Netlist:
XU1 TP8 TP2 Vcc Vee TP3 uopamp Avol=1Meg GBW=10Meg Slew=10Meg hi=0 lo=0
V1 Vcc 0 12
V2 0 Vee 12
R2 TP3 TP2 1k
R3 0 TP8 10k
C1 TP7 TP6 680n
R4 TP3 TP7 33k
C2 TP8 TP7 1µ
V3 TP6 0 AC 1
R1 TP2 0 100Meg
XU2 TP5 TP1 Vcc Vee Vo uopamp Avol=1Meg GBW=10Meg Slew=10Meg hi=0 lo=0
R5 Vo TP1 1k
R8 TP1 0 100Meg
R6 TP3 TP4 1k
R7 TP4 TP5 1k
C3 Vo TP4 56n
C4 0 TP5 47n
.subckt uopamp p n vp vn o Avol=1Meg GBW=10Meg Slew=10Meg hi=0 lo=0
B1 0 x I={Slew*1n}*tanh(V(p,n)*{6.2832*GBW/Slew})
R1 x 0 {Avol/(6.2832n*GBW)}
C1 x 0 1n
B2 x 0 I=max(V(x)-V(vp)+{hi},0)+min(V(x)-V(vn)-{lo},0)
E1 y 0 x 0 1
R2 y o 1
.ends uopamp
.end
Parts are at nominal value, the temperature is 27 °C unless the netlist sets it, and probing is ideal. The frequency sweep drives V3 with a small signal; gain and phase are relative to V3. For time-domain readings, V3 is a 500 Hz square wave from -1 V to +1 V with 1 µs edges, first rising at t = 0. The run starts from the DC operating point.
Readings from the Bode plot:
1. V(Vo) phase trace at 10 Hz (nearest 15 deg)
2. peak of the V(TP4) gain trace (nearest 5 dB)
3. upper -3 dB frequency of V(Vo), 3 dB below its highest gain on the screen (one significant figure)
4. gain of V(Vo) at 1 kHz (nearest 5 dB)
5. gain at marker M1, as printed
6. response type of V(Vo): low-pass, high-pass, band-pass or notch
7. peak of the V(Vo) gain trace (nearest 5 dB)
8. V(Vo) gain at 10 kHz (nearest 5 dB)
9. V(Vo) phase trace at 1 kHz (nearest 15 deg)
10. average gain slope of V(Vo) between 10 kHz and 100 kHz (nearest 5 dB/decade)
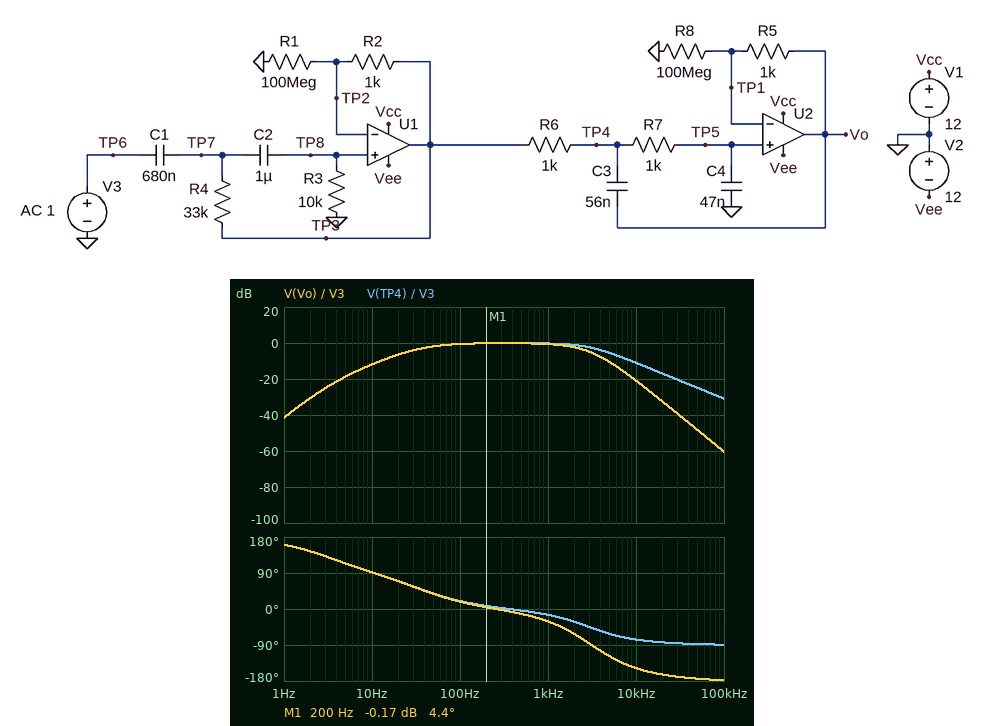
90 deg
0 dB
2 kHz
0 dB
-0.17 dB
band-pass
0 dB
-20 dB
-30 deg
-40 dB/decade
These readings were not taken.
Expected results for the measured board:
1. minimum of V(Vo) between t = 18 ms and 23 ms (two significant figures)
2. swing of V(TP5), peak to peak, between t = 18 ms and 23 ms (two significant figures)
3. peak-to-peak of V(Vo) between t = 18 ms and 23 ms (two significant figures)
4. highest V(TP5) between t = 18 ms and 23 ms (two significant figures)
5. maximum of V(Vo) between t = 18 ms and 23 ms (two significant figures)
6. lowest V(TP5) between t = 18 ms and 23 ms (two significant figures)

-1.1 V
2.1 V
2.1 V
1.0 V
1.0 V
-1.1 V
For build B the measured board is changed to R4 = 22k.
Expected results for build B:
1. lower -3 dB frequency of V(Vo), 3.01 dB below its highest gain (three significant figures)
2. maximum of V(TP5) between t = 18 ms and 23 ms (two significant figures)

34.2 Hz
990 mV
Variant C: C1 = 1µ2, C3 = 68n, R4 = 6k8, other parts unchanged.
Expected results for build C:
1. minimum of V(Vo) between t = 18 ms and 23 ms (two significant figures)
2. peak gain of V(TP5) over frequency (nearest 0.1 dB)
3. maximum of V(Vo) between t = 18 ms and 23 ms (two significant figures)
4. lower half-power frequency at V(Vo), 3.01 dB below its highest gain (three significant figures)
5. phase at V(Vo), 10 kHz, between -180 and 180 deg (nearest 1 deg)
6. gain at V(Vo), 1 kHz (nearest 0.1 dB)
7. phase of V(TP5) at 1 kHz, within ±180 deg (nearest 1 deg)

-1.2 V
0 dB
910 mV
21.0 Hz
-153 deg
-0.5 dB
-32 deg
